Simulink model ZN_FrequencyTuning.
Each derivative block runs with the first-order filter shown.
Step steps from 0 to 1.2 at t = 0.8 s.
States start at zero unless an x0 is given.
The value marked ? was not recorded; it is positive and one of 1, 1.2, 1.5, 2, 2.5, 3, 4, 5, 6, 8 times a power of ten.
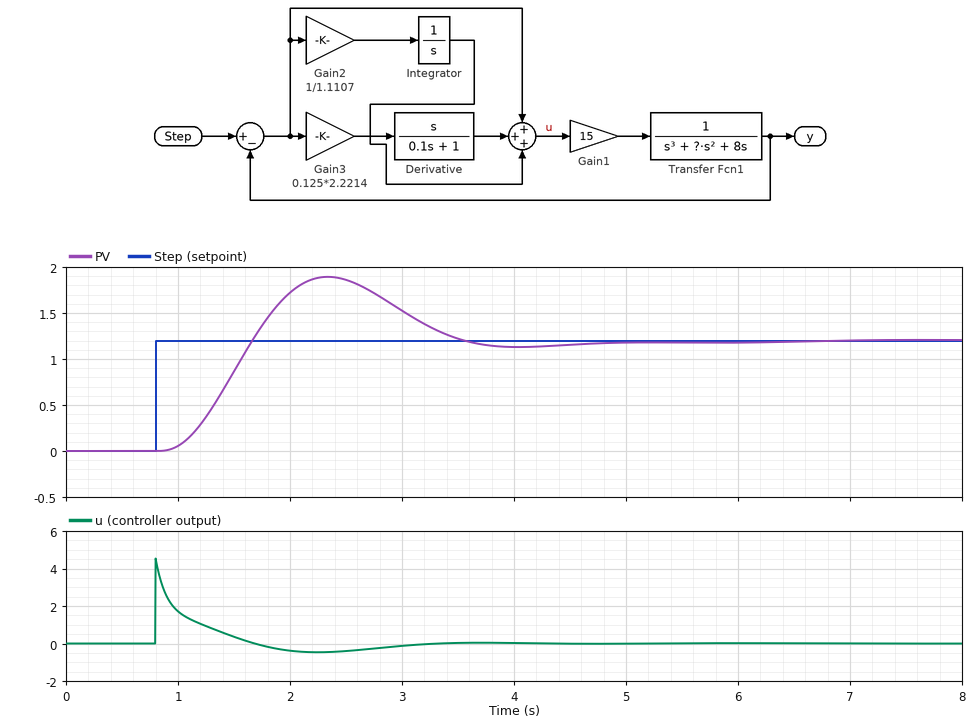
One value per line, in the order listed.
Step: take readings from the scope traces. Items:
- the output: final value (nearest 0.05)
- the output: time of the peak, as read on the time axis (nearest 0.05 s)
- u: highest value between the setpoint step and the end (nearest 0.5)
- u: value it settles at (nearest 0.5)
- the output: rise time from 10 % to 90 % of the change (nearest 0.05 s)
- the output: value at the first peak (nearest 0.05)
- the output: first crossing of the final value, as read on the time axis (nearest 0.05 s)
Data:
1.20
2.35 s
4.5
0.0
0.55 s
1.90
1.65 s
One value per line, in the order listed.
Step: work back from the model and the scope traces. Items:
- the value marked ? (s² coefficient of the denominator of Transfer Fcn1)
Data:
4
